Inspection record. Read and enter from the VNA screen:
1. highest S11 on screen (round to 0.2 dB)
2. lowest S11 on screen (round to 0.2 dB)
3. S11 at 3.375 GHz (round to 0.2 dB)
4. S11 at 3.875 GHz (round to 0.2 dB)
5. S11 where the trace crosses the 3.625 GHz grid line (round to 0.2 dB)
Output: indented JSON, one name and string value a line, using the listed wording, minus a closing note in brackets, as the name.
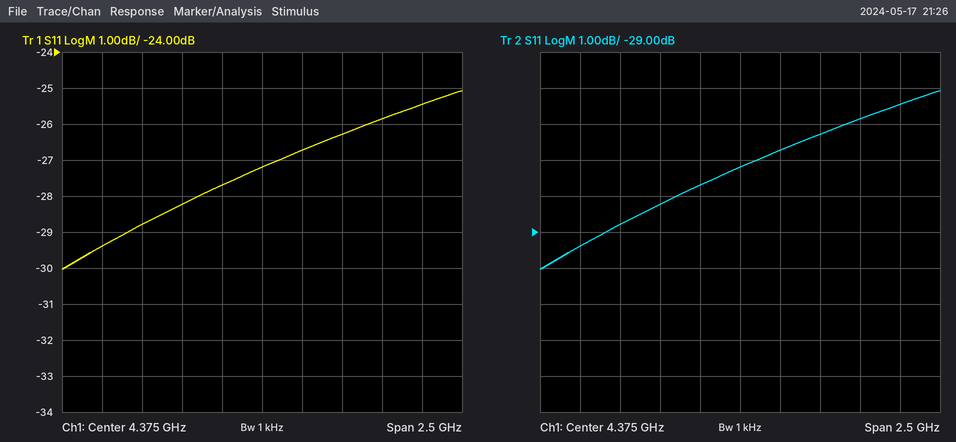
{
  "highest S11 on screen": "-25.0 dB",
  "lowest S11 on screen": "-30.0 dB",
  "S11 at 3.375 GHz": "-29.4 dB",
  "S11 at 3.875 GHz": "-28.2 dB",
  "S11 where the trace crosses the 3.625 GHz grid line": "-28.8 dB"
}
